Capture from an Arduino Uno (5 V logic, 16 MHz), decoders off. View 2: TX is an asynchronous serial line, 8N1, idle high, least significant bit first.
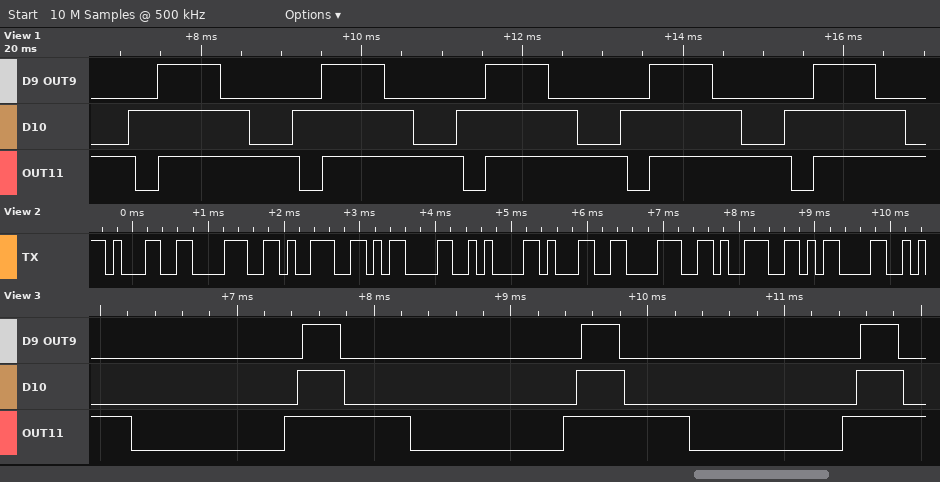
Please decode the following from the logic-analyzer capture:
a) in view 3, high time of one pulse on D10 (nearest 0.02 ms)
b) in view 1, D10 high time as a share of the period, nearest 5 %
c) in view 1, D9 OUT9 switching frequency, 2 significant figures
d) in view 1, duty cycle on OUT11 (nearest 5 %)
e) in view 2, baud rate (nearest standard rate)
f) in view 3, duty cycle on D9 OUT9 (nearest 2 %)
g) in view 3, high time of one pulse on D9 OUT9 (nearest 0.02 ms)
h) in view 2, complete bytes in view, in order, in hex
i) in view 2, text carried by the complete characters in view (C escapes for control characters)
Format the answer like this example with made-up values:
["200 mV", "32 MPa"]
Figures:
["0.34 ms", "75 %", "490 Hz", "85 %", "9600 baud", "14 %", "0.28 ms", "31 38 39 0D 0A 31 38 39 0D", "\"189\\r\\n189\\r\""]
